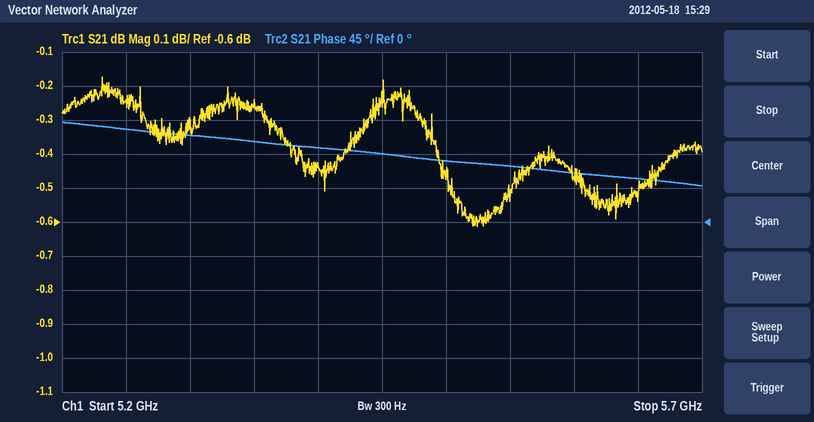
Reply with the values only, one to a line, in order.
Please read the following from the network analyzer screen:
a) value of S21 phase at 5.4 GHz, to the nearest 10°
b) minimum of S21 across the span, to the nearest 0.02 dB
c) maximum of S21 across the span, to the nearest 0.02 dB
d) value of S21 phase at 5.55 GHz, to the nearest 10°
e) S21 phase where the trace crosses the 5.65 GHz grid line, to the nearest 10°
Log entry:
100°
-0.62 dB
-0.18 dB
70°
60°
